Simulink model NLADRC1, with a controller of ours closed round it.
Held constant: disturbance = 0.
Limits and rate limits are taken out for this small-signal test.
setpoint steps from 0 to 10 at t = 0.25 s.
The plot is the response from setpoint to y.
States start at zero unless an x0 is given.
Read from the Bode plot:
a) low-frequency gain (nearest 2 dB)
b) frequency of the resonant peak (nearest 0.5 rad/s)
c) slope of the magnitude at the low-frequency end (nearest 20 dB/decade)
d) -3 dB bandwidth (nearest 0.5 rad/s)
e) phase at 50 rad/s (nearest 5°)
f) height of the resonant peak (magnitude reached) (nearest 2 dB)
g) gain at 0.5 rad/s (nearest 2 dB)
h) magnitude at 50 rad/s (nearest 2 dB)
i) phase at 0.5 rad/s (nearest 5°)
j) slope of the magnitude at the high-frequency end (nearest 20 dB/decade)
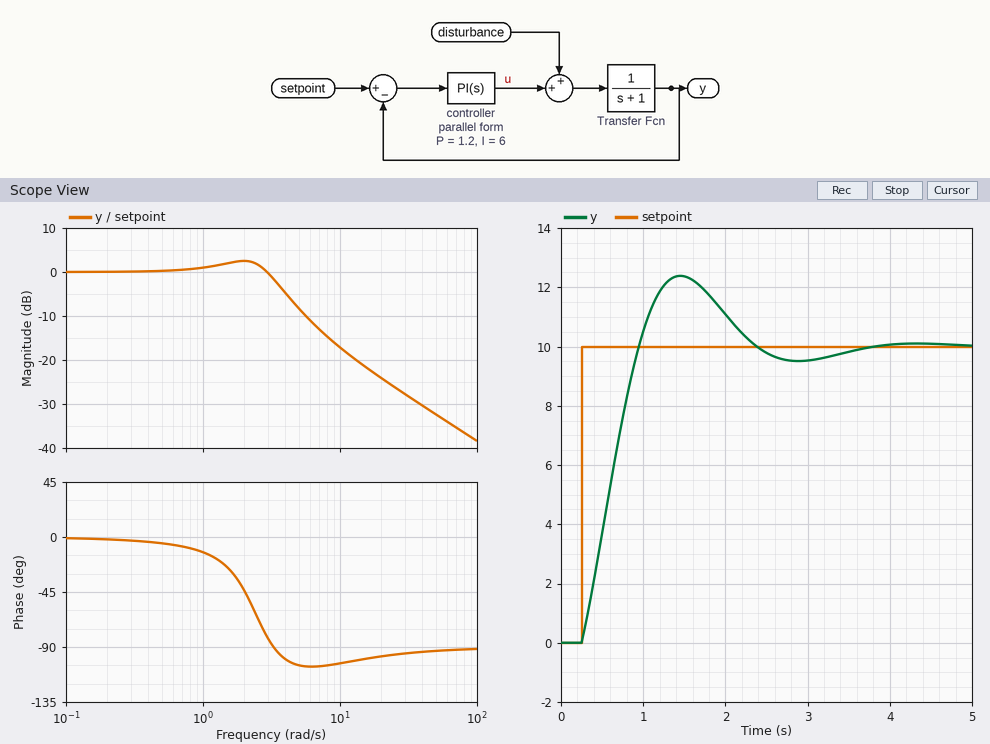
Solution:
0 dB
2.0 rad/s
0 dB/decade
3.5 rad/s
-95°
2 dB
0 dB
-32 dB
-5°
-20 dB/decade
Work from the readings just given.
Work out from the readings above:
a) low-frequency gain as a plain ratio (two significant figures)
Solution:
1.0
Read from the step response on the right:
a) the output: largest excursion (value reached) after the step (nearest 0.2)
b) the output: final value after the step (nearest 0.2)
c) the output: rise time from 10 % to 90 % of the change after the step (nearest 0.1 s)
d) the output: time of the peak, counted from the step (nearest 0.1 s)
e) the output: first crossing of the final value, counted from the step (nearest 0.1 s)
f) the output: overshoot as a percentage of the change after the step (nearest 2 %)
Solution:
12.4
10.0
0.5 s
1.2 s
0.7 s
24 %
